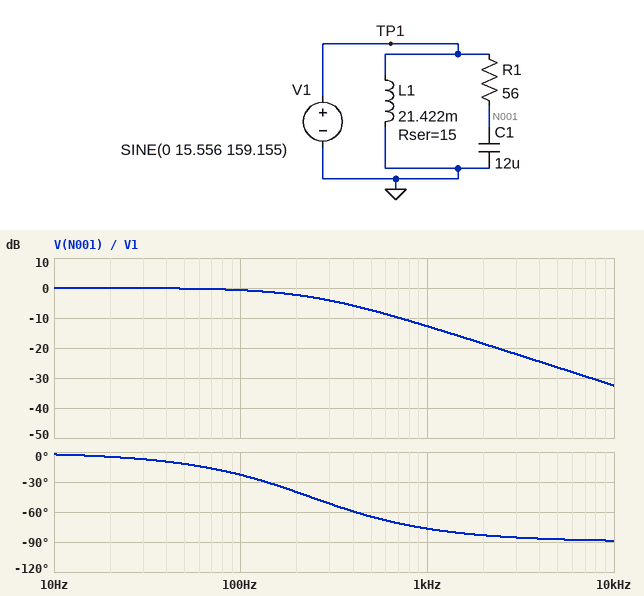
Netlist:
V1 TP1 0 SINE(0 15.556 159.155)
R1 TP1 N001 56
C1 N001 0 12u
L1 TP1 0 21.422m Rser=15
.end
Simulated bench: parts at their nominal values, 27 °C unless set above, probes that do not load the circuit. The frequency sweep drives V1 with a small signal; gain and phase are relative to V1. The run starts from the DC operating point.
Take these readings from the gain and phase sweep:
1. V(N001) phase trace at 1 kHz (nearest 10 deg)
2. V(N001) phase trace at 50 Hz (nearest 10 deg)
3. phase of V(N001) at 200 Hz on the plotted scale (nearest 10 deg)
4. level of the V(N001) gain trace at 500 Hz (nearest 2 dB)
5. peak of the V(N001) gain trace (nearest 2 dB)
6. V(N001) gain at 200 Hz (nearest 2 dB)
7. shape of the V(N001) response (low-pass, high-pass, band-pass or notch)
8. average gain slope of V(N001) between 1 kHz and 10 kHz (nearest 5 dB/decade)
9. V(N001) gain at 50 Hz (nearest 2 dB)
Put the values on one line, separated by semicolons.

-80 deg; -10 deg; -40 deg; -8 dB; 0 dB; -2 dB; low-pass; -20 dB/decade; 0 dB
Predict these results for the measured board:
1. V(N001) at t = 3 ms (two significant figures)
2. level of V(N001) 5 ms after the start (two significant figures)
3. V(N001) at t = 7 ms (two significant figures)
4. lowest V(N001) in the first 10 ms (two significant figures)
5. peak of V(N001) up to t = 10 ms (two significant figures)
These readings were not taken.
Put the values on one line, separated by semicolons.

8.7 V; -12 V; 1.6 V; -13 V; 13 V
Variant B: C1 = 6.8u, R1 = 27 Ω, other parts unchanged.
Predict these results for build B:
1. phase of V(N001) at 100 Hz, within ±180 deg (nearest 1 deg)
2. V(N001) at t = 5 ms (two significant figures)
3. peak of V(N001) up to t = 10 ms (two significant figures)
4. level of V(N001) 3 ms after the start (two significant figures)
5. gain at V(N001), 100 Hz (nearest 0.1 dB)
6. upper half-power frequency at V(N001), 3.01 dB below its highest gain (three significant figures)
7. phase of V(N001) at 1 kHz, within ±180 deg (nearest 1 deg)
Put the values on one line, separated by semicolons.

-7 deg; -15 V; 15 V; 4.9 V; -0.1 dB; 867 Hz; -49 deg
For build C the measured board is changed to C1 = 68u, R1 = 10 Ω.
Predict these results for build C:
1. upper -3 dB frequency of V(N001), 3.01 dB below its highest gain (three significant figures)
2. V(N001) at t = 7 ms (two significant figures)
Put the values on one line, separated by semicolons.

234 Hz; 1.5 V
